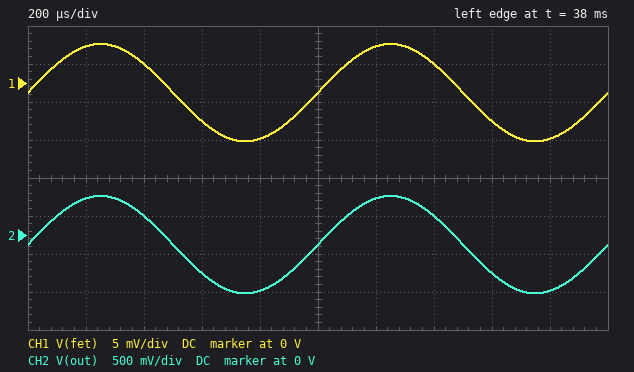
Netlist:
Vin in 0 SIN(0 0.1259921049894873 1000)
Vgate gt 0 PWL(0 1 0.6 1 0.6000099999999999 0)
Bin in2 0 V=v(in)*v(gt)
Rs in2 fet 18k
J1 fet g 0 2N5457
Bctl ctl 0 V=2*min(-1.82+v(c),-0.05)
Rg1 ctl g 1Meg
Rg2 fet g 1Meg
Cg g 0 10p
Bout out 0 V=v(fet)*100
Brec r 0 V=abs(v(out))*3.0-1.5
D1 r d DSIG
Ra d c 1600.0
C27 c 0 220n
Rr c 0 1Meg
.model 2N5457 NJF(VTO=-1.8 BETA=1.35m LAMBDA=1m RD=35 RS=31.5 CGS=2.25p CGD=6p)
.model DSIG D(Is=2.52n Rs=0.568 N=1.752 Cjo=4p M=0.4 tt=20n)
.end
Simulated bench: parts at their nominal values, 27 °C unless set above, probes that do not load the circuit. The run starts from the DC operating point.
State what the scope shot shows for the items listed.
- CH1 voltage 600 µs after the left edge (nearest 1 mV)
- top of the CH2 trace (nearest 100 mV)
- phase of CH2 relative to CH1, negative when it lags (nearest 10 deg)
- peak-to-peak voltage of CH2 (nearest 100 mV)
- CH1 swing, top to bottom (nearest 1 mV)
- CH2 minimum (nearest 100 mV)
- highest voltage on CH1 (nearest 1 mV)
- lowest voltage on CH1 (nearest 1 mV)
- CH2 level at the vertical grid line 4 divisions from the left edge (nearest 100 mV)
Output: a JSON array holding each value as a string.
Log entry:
["-5 mV", "500 mV", "0 deg", "1.3 V", "13 mV", "-800 mV", "5 mV", "-8 mV", "-700 mV"]
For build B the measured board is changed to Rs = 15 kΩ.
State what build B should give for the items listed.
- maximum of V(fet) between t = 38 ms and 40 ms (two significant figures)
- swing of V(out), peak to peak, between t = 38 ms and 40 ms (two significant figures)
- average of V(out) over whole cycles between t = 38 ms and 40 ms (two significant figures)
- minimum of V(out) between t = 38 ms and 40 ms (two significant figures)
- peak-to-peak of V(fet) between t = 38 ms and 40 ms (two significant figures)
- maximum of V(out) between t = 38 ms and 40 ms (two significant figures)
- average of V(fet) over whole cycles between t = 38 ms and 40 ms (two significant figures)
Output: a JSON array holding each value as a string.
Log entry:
["5.7 mV", "1.4 V", "-110 mV", "-790 mV", "14 mV", "570 mV", "-1.1 mV"]
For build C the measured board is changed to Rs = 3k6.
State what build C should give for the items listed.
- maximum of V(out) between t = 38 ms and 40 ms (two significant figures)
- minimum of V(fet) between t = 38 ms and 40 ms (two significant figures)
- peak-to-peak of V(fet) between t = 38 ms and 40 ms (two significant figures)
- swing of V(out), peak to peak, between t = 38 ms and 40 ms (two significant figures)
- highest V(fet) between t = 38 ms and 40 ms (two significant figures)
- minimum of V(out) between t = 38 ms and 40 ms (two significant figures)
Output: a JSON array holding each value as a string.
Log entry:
["1.1 V", "-11 mV", "22 mV", "2.2 V", "11 mV", "-1.1 V"]
